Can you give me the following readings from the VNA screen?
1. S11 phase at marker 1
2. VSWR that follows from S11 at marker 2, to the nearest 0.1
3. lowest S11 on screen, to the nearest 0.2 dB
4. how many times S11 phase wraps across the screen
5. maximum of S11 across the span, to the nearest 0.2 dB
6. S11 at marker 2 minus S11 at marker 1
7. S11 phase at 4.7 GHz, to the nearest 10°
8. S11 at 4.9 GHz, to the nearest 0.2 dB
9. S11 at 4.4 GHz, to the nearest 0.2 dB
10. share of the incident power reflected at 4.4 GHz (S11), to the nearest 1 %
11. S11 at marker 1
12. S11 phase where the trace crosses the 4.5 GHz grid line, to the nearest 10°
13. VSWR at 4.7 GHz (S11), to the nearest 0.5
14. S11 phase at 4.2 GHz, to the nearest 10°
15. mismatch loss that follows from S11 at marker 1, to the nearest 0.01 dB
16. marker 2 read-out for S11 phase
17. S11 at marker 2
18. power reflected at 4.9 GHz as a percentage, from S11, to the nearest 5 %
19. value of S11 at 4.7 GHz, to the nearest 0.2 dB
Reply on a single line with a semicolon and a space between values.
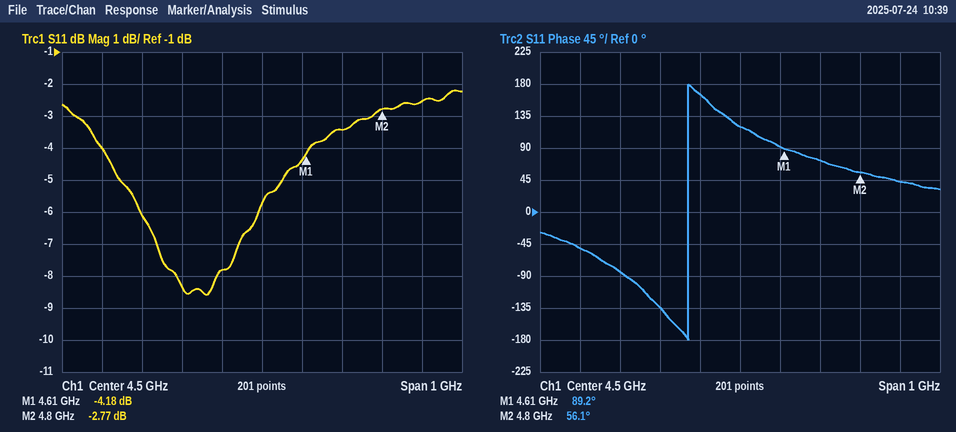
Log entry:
89.2°; 6.3; -8.6 dB; 1; -2.2 dB; 1.41 dB; 70°; -2.6 dB; -7.8 dB; 17 %; -4.18 dB; 120°; 5.0; -80°; 2.09 dB; 56.1°; -2.77 dB; 55 %; -3.4 dB
